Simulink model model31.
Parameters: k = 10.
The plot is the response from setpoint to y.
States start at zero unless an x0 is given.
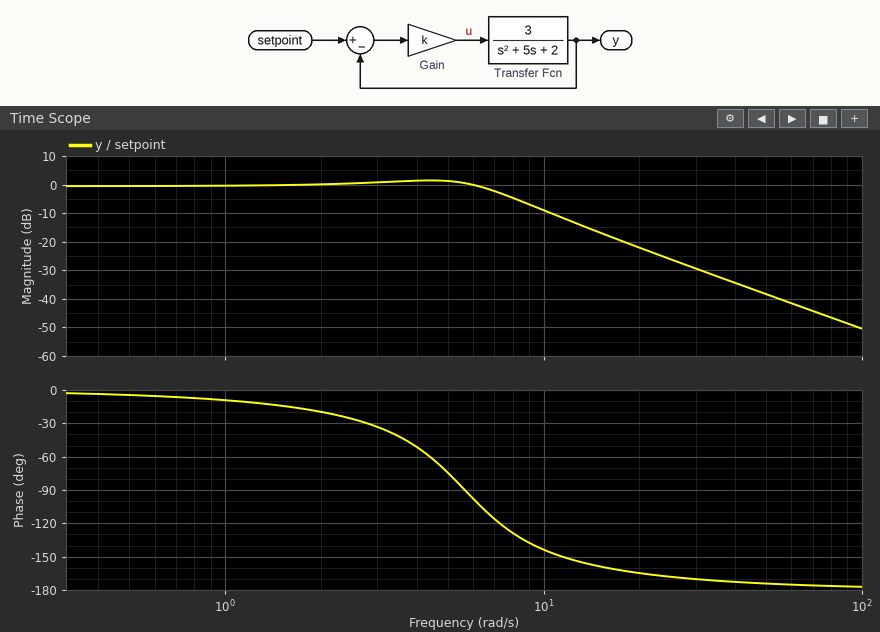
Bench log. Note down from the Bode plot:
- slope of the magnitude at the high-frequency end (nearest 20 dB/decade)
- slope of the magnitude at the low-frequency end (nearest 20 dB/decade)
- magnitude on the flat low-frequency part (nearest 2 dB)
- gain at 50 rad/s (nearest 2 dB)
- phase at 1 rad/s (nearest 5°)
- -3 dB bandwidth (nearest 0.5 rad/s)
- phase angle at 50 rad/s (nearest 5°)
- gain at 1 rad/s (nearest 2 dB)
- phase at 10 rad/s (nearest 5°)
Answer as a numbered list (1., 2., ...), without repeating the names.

1. -40 dB/decade
2. 0 dB/decade
3. 0 dB
4. -38 dB
5. -10°
6. 7.5 rad/s
7. -175°
8. 0 dB
9. -145°
